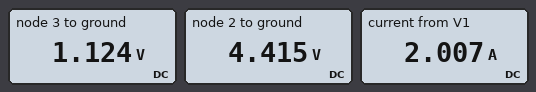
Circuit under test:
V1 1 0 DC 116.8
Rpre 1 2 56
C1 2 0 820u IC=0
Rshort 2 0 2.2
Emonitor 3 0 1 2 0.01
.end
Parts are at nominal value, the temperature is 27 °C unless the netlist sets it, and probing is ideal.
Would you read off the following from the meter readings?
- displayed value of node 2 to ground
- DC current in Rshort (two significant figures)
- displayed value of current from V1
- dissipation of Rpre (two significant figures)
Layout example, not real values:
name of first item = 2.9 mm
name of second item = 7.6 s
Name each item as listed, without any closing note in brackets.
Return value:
displayed value of node 2 to ground = 4.415 V
DC current in Rshort = 2.0 A
displayed value of current from V1 = 2.007 A
dissipation of Rpre = 230 W
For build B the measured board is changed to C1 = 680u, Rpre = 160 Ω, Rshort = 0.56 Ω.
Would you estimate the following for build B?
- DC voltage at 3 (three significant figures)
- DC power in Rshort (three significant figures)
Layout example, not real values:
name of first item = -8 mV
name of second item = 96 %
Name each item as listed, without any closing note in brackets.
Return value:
DC voltage at 3 = 1.16 V
DC power in Rshort = 296 mW
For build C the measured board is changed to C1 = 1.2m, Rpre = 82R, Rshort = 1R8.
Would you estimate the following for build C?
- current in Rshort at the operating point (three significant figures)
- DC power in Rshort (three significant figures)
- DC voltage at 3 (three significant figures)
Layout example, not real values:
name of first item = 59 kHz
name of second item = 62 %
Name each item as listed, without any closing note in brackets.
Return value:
current in Rshort at the operating point = 1.39 A
DC power in Rshort = 3.50 W
DC voltage at 3 = 1.14 V
